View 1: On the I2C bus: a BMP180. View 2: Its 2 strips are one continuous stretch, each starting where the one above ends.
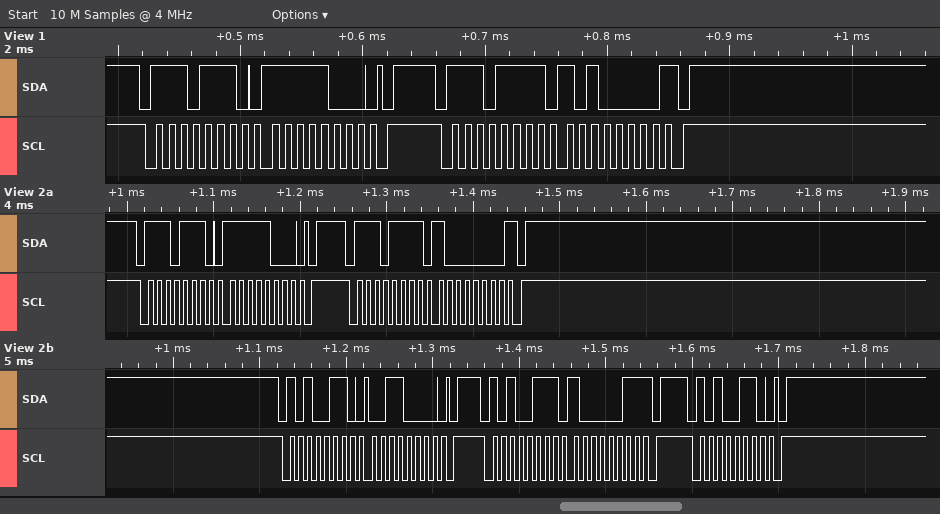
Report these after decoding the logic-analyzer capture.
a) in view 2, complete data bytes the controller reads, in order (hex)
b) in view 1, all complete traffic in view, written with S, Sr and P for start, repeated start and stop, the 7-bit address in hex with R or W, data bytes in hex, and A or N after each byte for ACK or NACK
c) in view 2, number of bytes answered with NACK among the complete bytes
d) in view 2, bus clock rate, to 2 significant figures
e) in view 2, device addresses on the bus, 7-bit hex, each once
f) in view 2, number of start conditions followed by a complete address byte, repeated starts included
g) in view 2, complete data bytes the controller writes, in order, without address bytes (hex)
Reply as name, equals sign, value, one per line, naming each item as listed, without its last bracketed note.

in view 2, complete data bytes the controller reads, in order = 80 83
in view 1, all complete traffic in view, written with S, Sr and P for start, repeated start and stop, the 7-bit address in hex with R or W, data bytes in hex, and A or N after each byte for ACK or NACK = S 77W A F8 A P S 77R A A0 N P
in view 2, number of bytes answered with NACK among the complete bytes = 2
in view 2, bus clock rate, to 2 significant figures = 100 kHz
in view 2, device addresses on the bus, 7-bit hex, each once = 0x77 0x53
in view 2, number of start conditions followed by a complete address byte, repeated starts included = 5
in view 2, complete data bytes the controller writes, in order, without address bytes = F8 30
